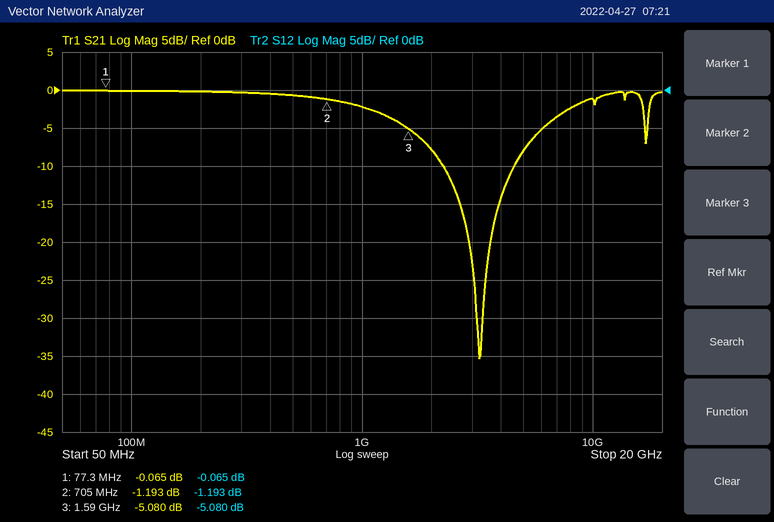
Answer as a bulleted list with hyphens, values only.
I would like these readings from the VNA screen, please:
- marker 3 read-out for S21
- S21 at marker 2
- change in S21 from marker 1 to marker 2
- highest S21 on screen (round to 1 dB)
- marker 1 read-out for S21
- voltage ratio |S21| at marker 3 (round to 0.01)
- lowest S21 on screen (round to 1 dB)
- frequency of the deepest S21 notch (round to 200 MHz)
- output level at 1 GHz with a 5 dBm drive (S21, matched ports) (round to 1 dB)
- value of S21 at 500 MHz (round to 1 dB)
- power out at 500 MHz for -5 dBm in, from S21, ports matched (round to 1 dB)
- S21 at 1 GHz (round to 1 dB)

- -5.080 dB
- -1.193 dB
- -1.128 dB
- 0 dB
- -0.065 dB
- 0.56
- -35 dB
- 3.2 GHz
- 3 dBm
- -1 dB
- -6 dBm
- -2 dB
